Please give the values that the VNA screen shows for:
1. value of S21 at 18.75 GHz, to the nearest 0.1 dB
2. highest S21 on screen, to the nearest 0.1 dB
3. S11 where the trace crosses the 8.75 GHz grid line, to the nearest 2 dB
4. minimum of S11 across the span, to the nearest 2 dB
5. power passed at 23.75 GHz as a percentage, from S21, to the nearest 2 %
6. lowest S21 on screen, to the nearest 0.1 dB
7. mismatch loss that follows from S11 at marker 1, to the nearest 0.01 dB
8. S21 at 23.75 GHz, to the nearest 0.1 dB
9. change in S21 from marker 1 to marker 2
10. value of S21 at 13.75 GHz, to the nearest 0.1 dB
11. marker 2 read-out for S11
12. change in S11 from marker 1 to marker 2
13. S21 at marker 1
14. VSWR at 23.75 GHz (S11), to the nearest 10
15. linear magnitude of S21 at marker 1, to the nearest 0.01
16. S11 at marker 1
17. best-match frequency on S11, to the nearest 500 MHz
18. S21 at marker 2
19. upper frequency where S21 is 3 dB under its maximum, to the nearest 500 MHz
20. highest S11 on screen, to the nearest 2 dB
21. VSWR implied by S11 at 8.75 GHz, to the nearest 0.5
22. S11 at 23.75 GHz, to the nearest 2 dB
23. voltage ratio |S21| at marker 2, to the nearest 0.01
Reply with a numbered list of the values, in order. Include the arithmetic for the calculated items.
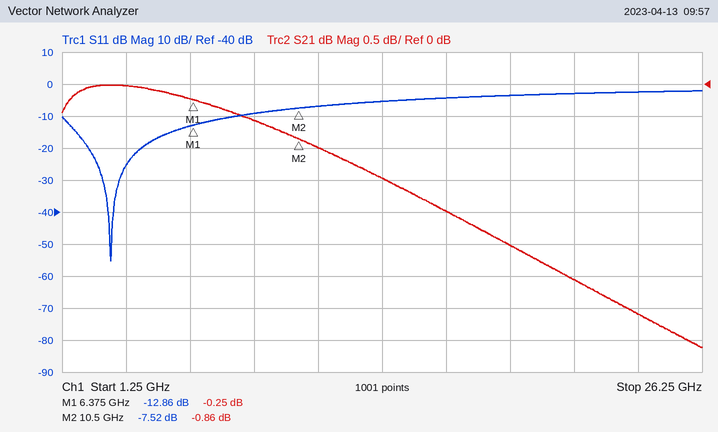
1. -2.5 dB
2. 0.0 dB
3. -10 dB
4. -56 dB
5. 10^(-3.6/10) ≈ 44 %
6. -4.1 dB
7. −10 log10(1 − 10^(-12.86/10)) ≈ 0.23 dB
8. -3.6 dB
9. -0.86 − (-0.25) = -0.61 dB
10. -1.5 dB
11. -7.52 dB
12. -7.52 − (-12.86) = 5.34 dB
13. -0.25 dB
14. |Γ| = 10^(-2/20) = 0.7943; VSWR = (1 + 0.7943)/(1 − 0.7943) ≈ 8.72, so 10 to the nearest 10
15. 10^(-0.25/20) ≈ 0.97
16. -12.86 dB
17. 3.0 GHz
18. -0.86 dB
19. 21.0 GHz
20. -2 dB
21. |Γ| = 10^(-10/20) = 0.3162; VSWR = (1 + 0.3162)/(1 − 0.3162) ≈ 1.92, so 2.0 to the nearest 0.5
22. -2 dB
23. 10^(-0.86/20) ≈ 0.91
